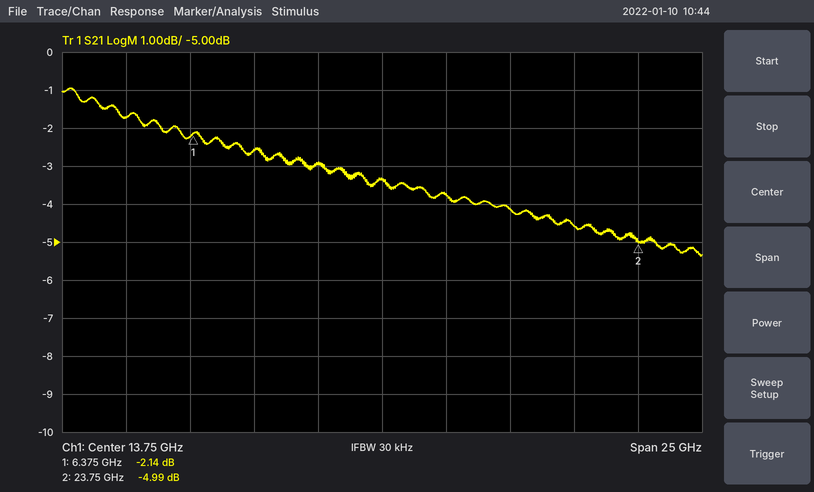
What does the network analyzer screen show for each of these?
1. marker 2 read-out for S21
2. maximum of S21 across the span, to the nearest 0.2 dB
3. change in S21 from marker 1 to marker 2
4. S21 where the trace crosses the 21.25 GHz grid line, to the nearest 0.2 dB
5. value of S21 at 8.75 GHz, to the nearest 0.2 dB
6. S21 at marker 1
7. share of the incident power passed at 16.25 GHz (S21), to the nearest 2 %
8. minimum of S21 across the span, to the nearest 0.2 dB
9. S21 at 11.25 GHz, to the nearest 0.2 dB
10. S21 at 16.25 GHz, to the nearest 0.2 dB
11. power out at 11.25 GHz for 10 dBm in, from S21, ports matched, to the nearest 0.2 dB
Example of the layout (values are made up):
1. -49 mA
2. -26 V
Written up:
1. -4.99 dB
2. -1.0 dB
3. -2.85 dB
4. -4.6 dB
5. -2.6 dB
6. -2.14 dB
7. 42 %
8. -5.4 dB
9. -3.0 dB
10. -3.8 dB
11. 7.0 dBm
